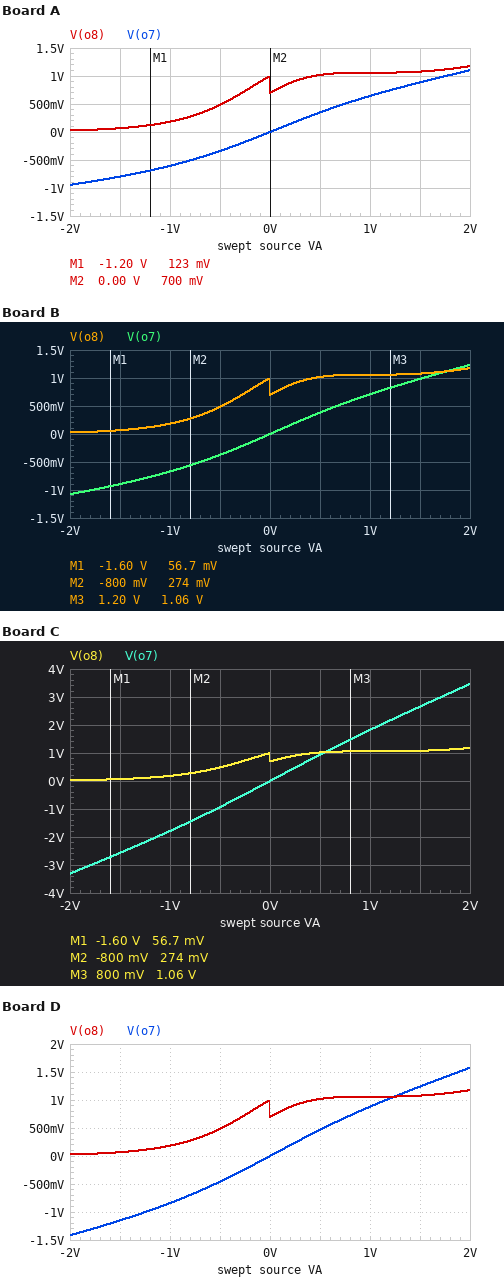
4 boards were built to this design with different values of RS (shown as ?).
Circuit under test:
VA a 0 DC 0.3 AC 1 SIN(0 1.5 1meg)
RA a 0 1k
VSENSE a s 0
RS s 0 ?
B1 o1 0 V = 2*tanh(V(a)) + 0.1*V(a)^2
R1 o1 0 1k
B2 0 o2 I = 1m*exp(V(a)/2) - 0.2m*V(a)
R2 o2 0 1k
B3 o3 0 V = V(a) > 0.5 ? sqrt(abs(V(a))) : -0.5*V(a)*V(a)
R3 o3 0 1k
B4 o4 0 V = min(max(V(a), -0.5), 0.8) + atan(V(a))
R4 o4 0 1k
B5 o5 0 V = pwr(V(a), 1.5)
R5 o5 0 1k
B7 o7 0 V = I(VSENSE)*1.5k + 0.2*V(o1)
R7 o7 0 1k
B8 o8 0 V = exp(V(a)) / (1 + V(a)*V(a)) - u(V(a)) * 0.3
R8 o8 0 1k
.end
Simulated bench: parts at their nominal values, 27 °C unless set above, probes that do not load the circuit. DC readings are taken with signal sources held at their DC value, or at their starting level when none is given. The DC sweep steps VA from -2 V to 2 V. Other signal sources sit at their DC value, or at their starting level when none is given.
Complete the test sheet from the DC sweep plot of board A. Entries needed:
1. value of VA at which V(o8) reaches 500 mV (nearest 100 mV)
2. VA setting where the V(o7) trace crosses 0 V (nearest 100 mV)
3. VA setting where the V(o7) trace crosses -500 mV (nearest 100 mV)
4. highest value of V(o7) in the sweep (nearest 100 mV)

-500 mV
0 V
-800 mV
1.1 V
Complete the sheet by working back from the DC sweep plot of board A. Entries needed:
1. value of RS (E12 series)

4.7 kΩ
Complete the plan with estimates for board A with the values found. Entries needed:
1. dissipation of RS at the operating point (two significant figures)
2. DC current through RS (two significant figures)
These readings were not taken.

19 µW
64 µA
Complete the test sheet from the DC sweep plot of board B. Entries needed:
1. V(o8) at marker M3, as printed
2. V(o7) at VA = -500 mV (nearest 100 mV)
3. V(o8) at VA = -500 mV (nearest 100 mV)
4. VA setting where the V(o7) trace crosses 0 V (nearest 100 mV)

1.06 V
-400 mV
500 mV
0 V
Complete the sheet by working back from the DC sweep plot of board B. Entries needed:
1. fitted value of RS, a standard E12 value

3.9 kΩ
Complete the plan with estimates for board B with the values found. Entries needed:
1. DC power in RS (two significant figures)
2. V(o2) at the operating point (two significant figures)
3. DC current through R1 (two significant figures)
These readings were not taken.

23 µW
1.1 V
590 µA
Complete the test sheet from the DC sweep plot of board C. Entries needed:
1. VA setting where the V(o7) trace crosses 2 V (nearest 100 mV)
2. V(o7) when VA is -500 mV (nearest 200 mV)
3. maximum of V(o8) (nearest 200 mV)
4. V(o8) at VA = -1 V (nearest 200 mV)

1.1 V
-1.0 V
1.2 V
200 mV
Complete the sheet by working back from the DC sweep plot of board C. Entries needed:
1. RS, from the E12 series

1 kΩ
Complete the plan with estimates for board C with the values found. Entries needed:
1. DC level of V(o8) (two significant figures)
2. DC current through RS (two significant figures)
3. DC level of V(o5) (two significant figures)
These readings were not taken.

940 mV
300 µA
160 mV
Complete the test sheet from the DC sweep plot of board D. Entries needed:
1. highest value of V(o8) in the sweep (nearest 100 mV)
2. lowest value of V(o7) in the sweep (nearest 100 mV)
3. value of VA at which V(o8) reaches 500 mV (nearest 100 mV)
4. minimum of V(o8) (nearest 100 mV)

1.2 V
-1.4 V
-500 mV
0 V
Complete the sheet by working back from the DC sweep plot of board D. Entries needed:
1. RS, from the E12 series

2.7 kΩ
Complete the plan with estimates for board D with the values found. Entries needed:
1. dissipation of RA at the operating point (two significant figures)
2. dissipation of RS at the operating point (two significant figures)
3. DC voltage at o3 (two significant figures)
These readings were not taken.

90 µW
33 µW
-45 mV
